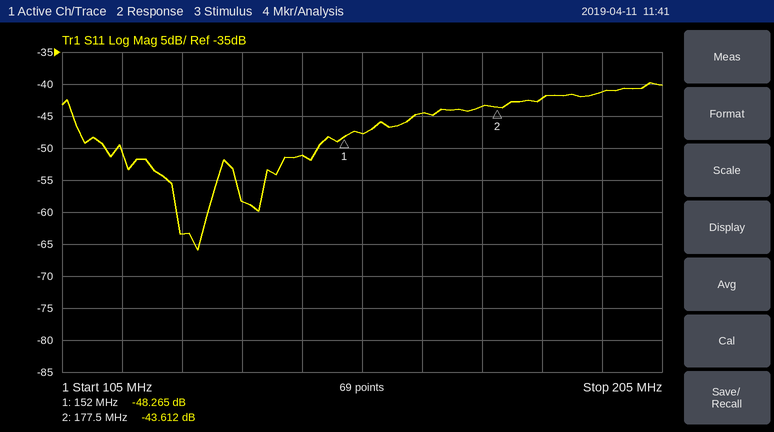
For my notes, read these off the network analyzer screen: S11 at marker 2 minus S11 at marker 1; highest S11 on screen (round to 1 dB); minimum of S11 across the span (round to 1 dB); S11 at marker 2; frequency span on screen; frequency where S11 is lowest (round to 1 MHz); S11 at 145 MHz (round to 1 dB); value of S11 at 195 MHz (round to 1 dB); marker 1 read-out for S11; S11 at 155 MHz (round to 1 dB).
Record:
4.653 dB
-40 dB
-66 dB
-43.612 dB
100 MHz
128 MHz
-51 dB
-41 dB
-48.265 dB
-48 dB
